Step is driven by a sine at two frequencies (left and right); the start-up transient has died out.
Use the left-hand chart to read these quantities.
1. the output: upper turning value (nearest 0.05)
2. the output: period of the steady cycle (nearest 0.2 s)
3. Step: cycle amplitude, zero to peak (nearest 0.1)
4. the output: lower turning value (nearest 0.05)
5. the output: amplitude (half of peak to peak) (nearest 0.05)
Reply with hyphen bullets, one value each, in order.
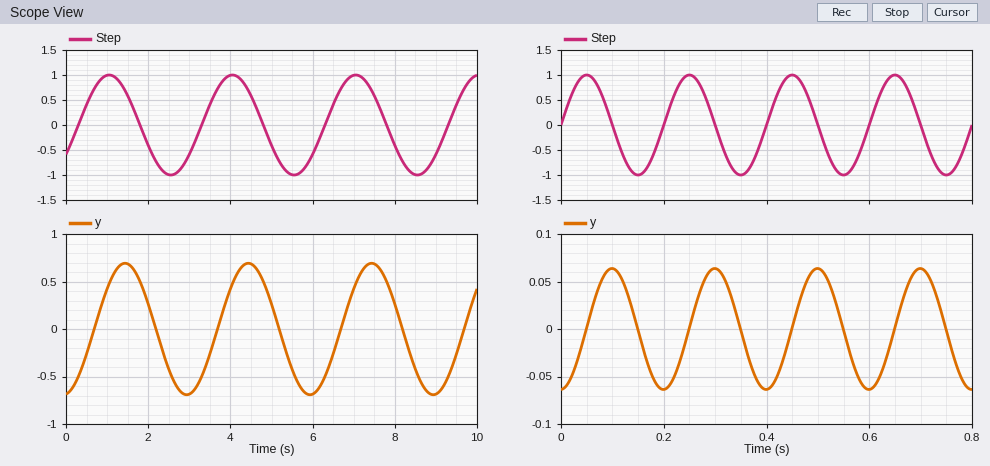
- 0.70
- 3.0 s
- 1.0
- -0.70
- 0.70
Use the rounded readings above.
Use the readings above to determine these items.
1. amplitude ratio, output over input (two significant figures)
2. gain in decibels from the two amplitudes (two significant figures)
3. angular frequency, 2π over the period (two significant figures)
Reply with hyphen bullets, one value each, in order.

- 0.70
- -3.1 dB
- 2.1 rad/s
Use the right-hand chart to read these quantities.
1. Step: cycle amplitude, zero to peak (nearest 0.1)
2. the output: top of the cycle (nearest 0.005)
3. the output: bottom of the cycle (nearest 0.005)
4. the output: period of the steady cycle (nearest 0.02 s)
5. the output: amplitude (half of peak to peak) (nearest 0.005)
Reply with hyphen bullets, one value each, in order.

- 1.0
- 0.065
- -0.065
- 0.20 s
- 0.065
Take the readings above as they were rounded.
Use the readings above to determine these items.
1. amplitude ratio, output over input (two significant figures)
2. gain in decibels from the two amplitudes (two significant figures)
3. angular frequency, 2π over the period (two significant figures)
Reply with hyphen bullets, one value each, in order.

- 0.065
- -24 dB
- 31 rad/s
